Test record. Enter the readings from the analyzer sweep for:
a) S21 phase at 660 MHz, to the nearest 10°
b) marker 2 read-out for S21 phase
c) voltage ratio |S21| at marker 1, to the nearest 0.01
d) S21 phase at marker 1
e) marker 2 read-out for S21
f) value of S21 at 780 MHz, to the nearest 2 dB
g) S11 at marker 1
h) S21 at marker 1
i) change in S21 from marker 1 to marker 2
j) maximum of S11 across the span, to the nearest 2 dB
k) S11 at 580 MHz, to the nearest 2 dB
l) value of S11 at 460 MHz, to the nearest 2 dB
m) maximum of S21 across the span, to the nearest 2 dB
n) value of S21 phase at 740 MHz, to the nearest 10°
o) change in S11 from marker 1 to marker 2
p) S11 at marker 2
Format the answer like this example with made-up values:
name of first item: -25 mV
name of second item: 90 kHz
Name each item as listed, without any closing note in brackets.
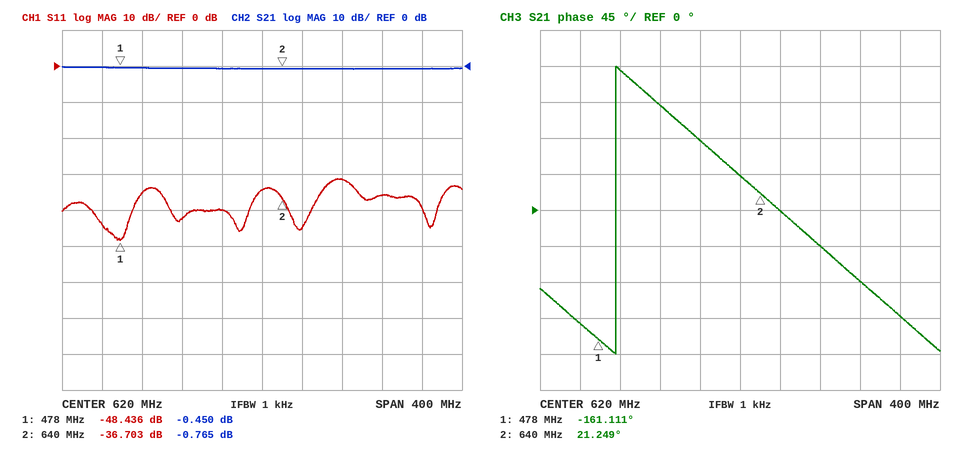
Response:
S21 phase at 660 MHz, to the nearest 10°: 0°
marker 2 read-out for S21 phase: 21.249°
voltage ratio |S21| at marker 1, to the nearest 0.01: 0.95
S21 phase at marker 1: -161.111°
marker 2 read-out for S21: -0.765 dB
value of S21 at 780 MHz, to the nearest 2 dB: 0 dB
S11 at marker 1: -48.436 dB
S21 at marker 1: -0.450 dB
change in S21 from marker 1 to marker 2: -0.315 dB
maximum of S11 across the span, to the nearest 2 dB: -32 dB
S11 at 580 MHz, to the nearest 2 dB: -40 dB
value of S11 at 460 MHz, to the nearest 2 dB: -44 dB
maximum of S21 across the span, to the nearest 2 dB: 0 dB
value of S21 phase at 740 MHz, to the nearest 10°: -90°
change in S11 from marker 1 to marker 2: 11.733 dB
S11 at marker 2: -36.703 dB
